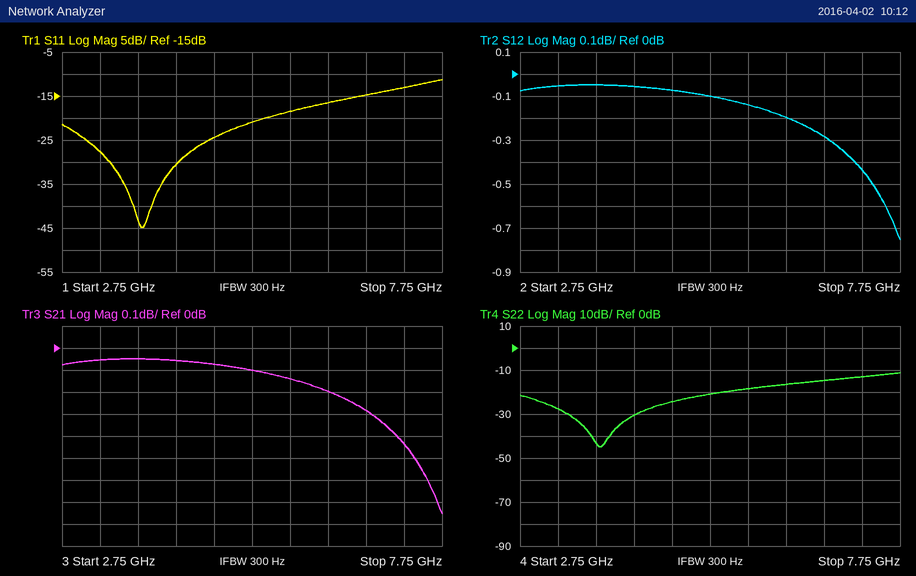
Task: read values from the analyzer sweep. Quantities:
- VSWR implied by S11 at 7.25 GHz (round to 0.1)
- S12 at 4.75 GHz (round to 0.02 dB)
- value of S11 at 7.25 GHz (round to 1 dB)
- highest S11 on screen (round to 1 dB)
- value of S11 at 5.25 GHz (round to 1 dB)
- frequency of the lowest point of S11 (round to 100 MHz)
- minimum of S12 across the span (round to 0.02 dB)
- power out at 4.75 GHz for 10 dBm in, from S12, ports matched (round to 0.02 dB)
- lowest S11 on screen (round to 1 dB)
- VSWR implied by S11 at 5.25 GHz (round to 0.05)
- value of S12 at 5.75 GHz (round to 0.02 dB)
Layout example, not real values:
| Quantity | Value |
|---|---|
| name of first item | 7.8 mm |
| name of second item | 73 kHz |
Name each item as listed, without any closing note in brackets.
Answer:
| Quantity | Value |
|---|---|
| VSWR implied by S11 at 7.25 GHz | 1.6 |
| S12 at 4.75 GHz | -0.08 dB |
| value of S11 at 7.25 GHz | -13 dB |
| highest S11 on screen | -11 dB |
| value of S11 at 5.25 GHz | -21 dB |
| frequency of the lowest point of S11 | 3.8 GHz |
| minimum of S12 across the span | -0.76 dB |
| power out at 4.75 GHz for 10 dBm in, from S12, ports matched | 9.92 dBm |
| lowest S11 on screen | -45 dB |
| VSWR implied by S11 at 5.25 GHz | 1.20 |
| value of S12 at 5.75 GHz | -0.14 dB |
